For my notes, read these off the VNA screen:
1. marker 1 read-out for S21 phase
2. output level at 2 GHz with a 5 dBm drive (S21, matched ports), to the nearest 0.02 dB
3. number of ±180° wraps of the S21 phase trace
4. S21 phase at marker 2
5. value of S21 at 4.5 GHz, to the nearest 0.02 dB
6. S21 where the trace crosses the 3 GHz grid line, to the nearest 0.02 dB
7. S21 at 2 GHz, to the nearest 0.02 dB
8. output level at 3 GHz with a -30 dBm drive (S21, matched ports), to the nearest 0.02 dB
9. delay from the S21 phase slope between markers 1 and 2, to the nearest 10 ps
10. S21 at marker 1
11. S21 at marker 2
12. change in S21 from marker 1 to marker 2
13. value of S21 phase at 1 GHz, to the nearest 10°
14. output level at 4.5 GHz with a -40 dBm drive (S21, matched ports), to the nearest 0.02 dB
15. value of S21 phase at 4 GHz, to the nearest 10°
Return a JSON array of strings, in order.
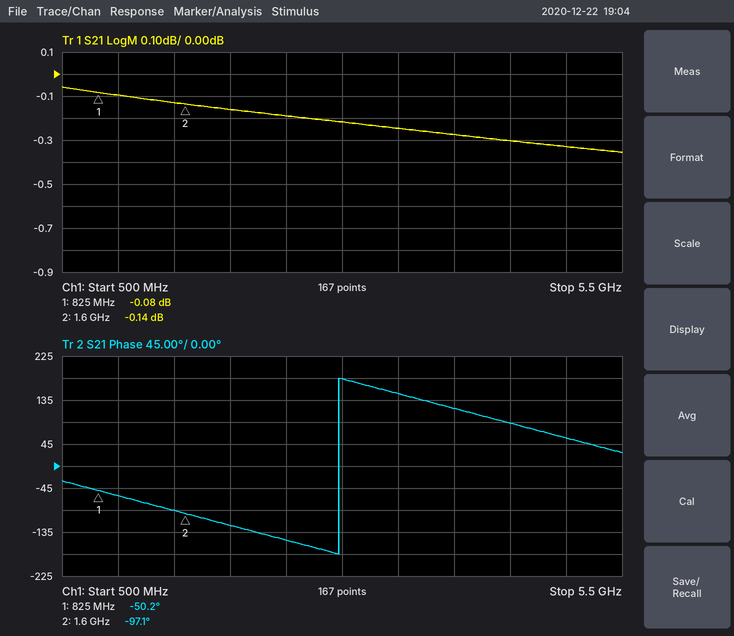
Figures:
["-50.2°", "4.84 dBm", "1", "-97.1°", "-0.30 dB", "-0.22 dB", "-0.16 dB", "-30.22 dBm", "170 ps", "-0.08 dB", "-0.14 dB", "-0.06 dB", "-60°", "-40.30 dBm", "120°"]
